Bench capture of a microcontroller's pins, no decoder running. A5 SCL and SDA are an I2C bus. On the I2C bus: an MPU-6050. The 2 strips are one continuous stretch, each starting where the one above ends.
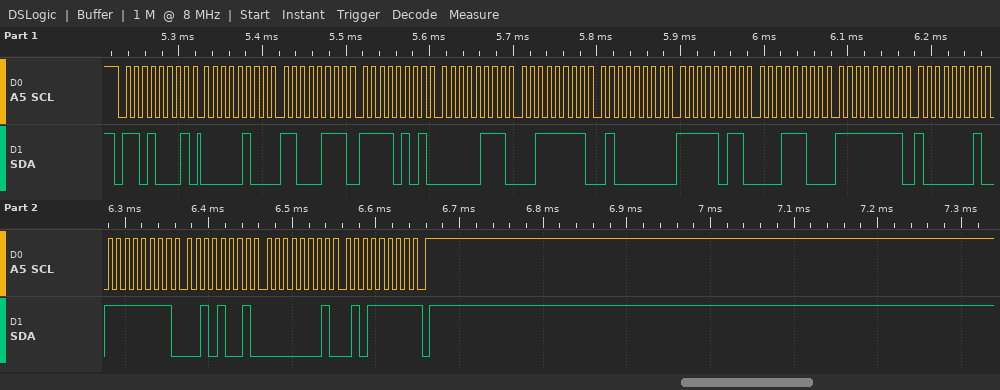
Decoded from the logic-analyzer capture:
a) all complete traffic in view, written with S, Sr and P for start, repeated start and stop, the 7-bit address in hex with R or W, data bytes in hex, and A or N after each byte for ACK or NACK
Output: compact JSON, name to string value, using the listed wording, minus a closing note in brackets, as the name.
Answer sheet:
{"all complete traffic in view, written with S, Sr and P for start, repeated start and stop, the 7-bit address in hex with R or W, data bytes in hex, and A or N after each byte for ACK or NACK": "S 68R A 04 A C7 A F5 A 07 A 3F A 40 A FB A 1C A FF A 81 A FF A 29 A 01 A 5F N P"}
